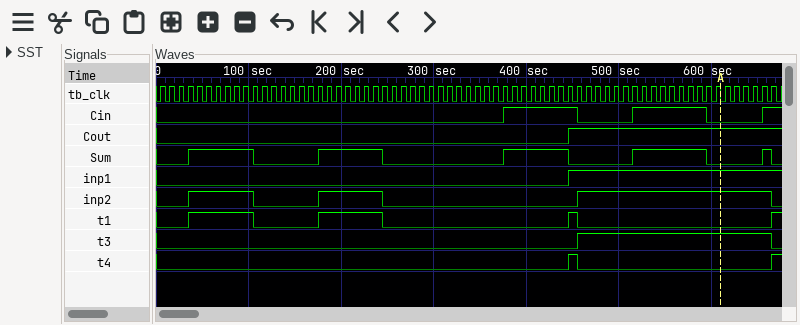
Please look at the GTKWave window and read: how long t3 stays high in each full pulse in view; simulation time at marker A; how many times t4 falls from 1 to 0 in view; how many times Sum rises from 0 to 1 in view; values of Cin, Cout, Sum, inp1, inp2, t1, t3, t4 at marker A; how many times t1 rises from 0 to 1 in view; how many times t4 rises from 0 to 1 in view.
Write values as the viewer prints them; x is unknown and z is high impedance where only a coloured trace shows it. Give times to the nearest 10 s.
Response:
210 s
610 s
1
5
Cin=0, Cout=1, Sum=0, inp1=1, inp2=1, t1=0, t3=1, t4=0
4
2
